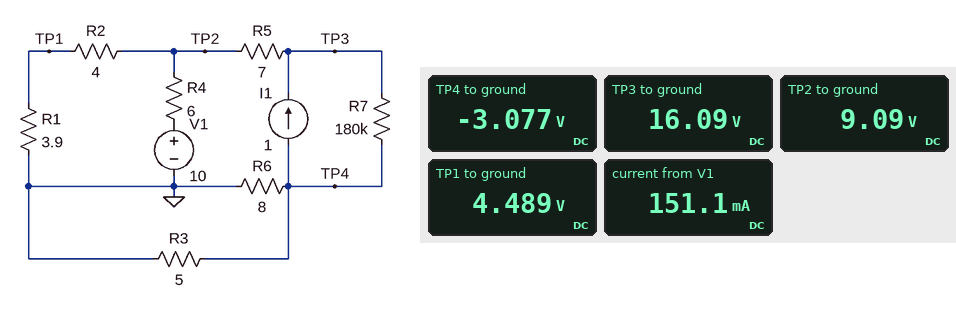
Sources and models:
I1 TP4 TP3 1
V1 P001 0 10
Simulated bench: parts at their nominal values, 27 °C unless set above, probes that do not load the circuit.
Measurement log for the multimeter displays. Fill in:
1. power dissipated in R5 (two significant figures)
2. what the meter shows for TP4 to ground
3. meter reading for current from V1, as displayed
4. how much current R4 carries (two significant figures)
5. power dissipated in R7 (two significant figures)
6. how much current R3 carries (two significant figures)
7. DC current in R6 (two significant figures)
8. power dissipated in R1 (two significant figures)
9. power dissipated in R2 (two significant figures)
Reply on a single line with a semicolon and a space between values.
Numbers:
7.0 W; -3.077 V; 151.1 mA; 150 mA; 2.0 mW; 620 mA; 380 mA; 5.2 W; 5.3 W
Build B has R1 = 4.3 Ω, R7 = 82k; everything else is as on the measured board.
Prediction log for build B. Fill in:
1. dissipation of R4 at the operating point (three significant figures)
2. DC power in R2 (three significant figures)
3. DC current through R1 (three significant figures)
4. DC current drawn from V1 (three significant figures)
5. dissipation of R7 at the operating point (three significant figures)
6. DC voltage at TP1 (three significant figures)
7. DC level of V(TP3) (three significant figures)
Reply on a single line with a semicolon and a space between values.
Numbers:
85.0 mW; 5.01 W; 1.12 A; 119 mA; 4.57 mW; 4.81 V; 16.3 V
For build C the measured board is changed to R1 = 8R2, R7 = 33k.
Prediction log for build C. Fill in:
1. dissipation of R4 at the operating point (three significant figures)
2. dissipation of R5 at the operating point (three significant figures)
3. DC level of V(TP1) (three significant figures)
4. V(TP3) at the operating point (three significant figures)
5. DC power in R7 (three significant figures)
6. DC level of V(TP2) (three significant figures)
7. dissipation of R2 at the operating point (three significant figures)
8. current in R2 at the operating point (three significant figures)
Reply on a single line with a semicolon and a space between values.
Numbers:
87.1 mW; 6.99 W; 7.21 V; 17.7 V; 13.1 mW; 10.7 V; 3.09 W; 879 mA
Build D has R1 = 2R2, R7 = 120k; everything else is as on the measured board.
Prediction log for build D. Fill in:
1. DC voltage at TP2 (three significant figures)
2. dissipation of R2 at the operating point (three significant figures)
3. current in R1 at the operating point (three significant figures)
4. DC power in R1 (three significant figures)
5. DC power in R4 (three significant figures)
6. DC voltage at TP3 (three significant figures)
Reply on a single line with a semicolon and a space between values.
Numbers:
8.13 V; 6.88 W; 1.31 A; 3.78 W; 582 mW; 15.1 V
